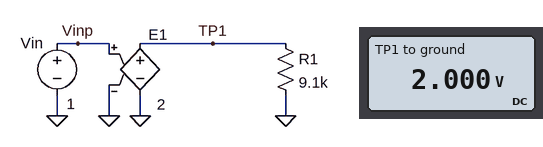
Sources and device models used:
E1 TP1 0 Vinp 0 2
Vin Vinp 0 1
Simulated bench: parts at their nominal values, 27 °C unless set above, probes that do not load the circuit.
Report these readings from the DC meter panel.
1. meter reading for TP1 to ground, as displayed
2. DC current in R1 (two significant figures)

2.000 V
220 µA
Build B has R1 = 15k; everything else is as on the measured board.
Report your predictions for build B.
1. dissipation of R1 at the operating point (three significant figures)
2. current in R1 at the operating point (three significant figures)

267 µW
133 µA
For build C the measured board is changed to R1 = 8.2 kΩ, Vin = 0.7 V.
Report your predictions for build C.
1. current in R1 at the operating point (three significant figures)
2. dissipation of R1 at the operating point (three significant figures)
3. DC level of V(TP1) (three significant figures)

171 µA
239 µW
1.40 V
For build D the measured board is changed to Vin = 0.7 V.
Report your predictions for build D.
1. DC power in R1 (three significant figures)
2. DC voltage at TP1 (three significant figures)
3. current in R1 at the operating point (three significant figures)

215 µW
1.40 V
154 µA
